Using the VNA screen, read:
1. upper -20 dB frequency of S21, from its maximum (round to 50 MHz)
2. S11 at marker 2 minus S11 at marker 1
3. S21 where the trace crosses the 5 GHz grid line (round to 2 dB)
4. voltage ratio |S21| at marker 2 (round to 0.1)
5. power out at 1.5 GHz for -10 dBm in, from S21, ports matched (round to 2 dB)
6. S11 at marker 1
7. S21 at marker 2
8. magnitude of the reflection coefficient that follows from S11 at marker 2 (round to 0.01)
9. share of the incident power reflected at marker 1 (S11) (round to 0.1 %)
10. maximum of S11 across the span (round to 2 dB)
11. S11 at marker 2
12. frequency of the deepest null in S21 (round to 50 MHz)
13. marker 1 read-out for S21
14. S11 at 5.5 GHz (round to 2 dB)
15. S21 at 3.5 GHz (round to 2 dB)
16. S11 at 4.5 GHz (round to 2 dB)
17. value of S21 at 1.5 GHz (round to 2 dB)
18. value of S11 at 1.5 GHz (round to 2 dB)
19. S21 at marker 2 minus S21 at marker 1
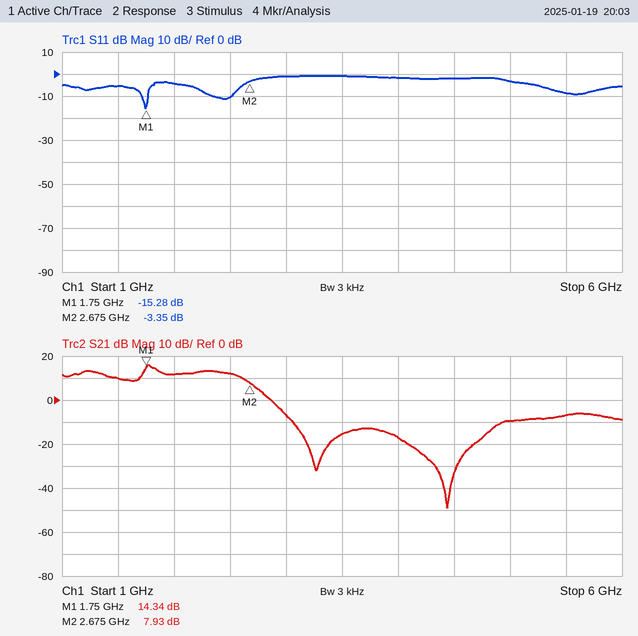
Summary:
2.95 GHz
11.93 dB
-10 dB
2.5
0 dBm
-15.28 dB
7.93 dB
0.68
3.0 %
0 dB
-3.35 dB
4.45 GHz
14.34 dB
-8 dB
-16 dB
-2 dB
10 dB
-6 dB
-6.41 dB
